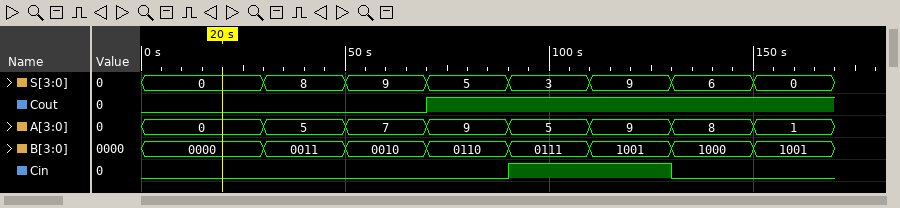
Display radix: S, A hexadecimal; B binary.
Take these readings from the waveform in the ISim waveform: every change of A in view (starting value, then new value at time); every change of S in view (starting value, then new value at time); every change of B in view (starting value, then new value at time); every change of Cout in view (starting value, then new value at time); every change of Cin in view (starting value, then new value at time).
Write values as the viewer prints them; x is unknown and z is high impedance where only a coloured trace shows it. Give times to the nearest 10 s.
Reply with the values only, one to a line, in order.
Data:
0, 5 at 30 s, 7 at 50 s, 9 at 70 s, 5 at 90 s, 9 at 110 s, 8 at 130 s, 1 at 150 s
0, 8 at 30 s, 9 at 50 s, 5 at 70 s, 3 at 90 s, 9 at 110 s, 6 at 130 s, 0 at 150 s
0000, 0011 at 30 s, 0010 at 50 s, 0110 at 70 s, 0111 at 90 s, 1001 at 110 s, 1000 at 130 s, 1001 at 150 s
0, 1 at 70 s
0, 1 at 90 s, 0 at 130 s
